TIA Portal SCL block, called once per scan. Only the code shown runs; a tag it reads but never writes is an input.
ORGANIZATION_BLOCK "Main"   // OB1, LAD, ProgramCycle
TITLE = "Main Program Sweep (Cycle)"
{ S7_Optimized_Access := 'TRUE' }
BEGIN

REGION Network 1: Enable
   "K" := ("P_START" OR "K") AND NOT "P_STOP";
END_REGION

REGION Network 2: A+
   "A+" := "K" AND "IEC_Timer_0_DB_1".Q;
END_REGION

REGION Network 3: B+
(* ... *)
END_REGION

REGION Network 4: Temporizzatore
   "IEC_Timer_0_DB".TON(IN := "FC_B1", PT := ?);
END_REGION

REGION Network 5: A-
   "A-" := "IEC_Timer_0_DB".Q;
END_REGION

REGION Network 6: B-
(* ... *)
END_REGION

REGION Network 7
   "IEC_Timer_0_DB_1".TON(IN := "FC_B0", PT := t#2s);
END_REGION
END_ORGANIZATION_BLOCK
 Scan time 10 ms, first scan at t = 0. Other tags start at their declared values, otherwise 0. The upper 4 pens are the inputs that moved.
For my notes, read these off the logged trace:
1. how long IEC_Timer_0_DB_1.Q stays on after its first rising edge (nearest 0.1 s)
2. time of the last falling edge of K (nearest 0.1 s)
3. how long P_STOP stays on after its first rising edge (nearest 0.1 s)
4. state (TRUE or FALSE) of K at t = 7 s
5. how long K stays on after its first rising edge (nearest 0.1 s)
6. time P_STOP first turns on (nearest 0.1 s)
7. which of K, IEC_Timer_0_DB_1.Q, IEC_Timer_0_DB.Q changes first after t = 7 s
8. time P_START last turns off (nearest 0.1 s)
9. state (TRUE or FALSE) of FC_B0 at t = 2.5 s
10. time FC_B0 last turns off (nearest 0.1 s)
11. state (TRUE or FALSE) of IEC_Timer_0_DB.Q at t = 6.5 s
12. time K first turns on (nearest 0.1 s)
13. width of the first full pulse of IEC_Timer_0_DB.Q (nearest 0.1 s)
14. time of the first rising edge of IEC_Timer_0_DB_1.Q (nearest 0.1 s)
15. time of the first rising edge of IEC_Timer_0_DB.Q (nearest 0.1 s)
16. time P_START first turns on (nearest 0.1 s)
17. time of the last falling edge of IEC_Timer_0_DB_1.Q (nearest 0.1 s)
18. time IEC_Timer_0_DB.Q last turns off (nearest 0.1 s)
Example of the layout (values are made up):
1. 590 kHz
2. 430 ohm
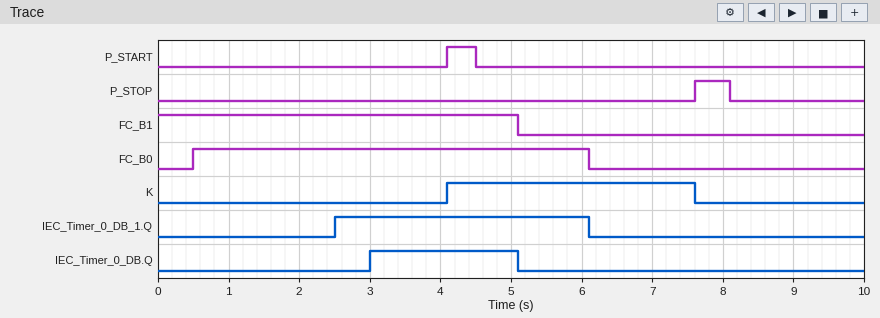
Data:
1. 3.6 s
2. 7.6 s
3. 0.5 s
4. TRUE
5. 3.5 s
6. 7.6 s
7. K
8. 4.5 s
9. TRUE
10. 6.1 s
11. FALSE
12. 4.1 s
13. 2.1 s
14. 2.5 s
15. 3.0 s
16. 4.1 s
17. 6.1 s
18. 5.1 s
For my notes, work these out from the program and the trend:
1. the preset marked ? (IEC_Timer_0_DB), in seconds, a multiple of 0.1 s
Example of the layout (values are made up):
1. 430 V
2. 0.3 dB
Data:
1. 3.0 s
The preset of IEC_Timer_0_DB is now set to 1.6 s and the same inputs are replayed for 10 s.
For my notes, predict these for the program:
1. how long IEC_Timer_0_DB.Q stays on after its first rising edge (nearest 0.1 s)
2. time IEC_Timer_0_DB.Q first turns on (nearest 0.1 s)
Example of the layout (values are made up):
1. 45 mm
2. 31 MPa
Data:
1. 3.5 s
2. 1.6 s
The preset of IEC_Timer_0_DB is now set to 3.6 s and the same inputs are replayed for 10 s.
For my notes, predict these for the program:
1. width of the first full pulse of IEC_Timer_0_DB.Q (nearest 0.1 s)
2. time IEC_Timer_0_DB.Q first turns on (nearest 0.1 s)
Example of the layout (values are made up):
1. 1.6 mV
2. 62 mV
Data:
1. 1.5 s
2. 3.6 s
